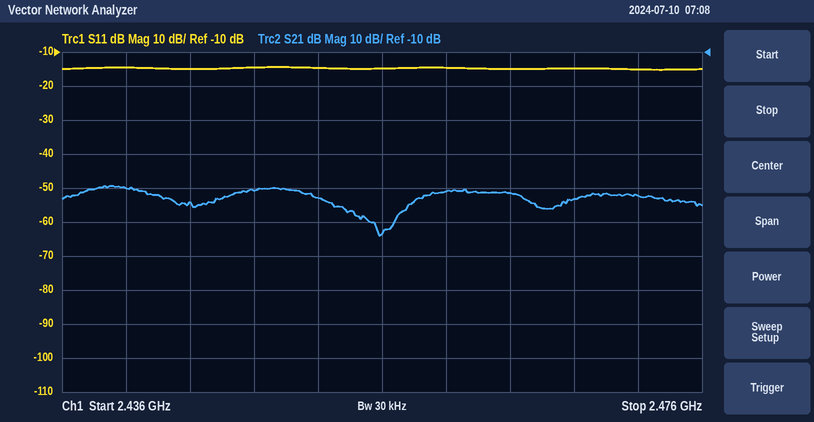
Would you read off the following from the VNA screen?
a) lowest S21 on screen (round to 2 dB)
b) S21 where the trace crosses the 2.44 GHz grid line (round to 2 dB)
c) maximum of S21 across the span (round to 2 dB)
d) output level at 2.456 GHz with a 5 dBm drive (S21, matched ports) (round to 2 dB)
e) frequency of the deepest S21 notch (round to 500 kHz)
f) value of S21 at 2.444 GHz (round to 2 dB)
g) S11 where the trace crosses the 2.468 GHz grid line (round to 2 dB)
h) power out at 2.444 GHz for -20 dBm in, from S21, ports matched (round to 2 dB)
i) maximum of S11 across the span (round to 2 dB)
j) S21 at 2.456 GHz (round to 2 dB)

-64 dB
-50 dB
-50 dB
-58 dBm
2.4560 GHz
-54 dB
-14 dB
-74 dBm
-14 dB
-64 dB
